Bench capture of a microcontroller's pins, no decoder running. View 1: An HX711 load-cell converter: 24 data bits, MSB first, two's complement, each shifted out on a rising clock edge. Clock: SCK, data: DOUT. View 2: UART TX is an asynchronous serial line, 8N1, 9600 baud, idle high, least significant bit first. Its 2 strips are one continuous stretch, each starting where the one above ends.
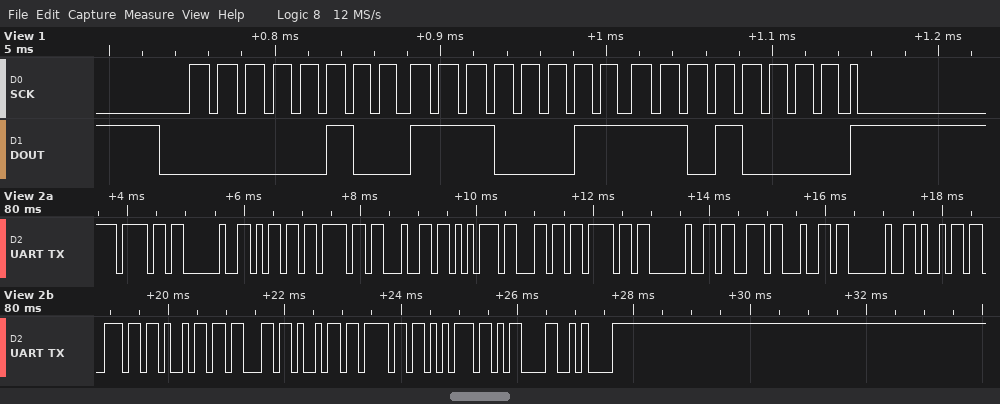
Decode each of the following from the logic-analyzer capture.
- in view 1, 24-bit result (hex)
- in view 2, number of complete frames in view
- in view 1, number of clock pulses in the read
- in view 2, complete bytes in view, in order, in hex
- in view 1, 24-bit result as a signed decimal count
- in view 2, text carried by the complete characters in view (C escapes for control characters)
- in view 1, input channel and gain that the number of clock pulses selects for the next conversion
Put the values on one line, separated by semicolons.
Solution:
0x04E3D0; 21; 25; 6F 20 6D 6F 64 75 6C 6F 20 73 64 20 69 6E 69 63 69 6F 75 0D 0A; 320464; "o modulo sd iniciou\r\n"; channel A, gain 128
